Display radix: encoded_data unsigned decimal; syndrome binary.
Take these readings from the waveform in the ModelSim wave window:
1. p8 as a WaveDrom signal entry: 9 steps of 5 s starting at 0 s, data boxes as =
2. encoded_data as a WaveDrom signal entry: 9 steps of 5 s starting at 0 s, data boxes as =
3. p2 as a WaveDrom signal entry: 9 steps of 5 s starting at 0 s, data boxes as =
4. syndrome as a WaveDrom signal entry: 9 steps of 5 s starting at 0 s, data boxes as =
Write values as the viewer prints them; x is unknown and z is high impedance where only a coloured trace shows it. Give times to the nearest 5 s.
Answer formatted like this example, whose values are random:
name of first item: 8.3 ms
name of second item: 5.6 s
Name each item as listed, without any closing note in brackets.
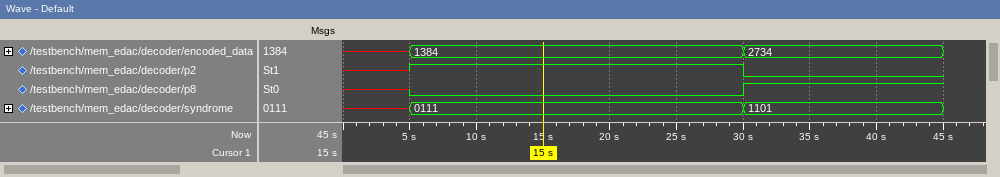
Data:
p8 as a WaveDrom signal entry: 9 steps of 5 s starting at 0 s, data boxes as =: {name: 'p8', wave: 'x0....1..'}
encoded_data as a WaveDrom signal entry: 9 steps of 5 s starting at 0 s, data boxes as =: {name: 'encoded_data', wave: 'x=....=..', data: '1384 2734'}
p2 as a WaveDrom signal entry: 9 steps of 5 s starting at 0 s, data boxes as =: {name: 'p2', wave: 'x1....0..'}
syndrome as a WaveDrom signal entry: 9 steps of 5 s starting at 0 s, data boxes as =: {name: 'syndrome', wave: 'x=....=..', data: '0111 1101'}
